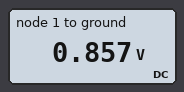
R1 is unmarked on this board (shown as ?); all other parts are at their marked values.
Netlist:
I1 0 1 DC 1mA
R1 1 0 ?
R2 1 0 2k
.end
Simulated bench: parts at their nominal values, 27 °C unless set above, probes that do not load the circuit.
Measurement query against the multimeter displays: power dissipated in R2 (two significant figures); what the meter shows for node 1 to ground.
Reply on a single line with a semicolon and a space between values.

370 µW; 0.857 V
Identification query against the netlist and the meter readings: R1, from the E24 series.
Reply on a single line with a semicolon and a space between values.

1.5 kΩ
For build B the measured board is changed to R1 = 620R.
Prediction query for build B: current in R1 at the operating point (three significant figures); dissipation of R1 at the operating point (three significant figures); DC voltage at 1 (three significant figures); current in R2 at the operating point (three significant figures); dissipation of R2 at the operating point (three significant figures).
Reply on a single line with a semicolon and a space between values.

763 µA; 361 µW; 473 mV; 237 µA; 112 µW
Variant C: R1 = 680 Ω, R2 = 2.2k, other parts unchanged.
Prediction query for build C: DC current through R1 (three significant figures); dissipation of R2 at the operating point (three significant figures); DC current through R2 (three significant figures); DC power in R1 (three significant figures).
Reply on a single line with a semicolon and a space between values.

764 µA; 123 µW; 236 µA; 397 µW
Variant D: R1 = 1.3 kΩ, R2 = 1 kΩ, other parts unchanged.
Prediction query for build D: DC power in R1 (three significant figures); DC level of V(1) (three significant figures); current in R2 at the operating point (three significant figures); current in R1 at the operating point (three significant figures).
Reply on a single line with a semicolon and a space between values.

246 µW; 565 mV; 565 µA; 435 µA
